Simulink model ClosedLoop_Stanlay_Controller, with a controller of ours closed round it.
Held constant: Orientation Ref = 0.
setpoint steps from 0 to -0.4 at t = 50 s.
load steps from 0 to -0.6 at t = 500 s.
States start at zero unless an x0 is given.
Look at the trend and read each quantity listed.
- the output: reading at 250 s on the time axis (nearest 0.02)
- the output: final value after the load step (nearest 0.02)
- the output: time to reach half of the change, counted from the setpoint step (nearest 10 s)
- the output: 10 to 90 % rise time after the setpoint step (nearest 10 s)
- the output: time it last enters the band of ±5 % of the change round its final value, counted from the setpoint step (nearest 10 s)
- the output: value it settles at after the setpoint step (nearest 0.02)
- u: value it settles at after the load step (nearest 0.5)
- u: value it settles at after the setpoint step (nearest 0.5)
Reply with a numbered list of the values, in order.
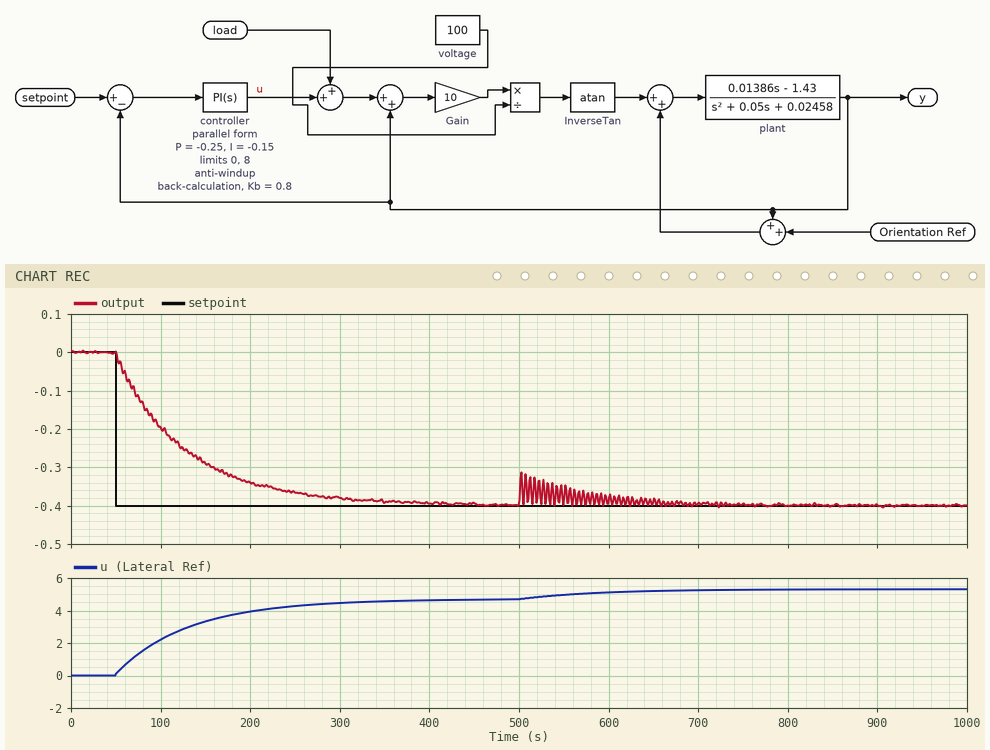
1. -0.36
2. -0.40
3. 50 s
4. 180 s
5. 250 s
6. -0.40
7. 5.5
8. 4.5
